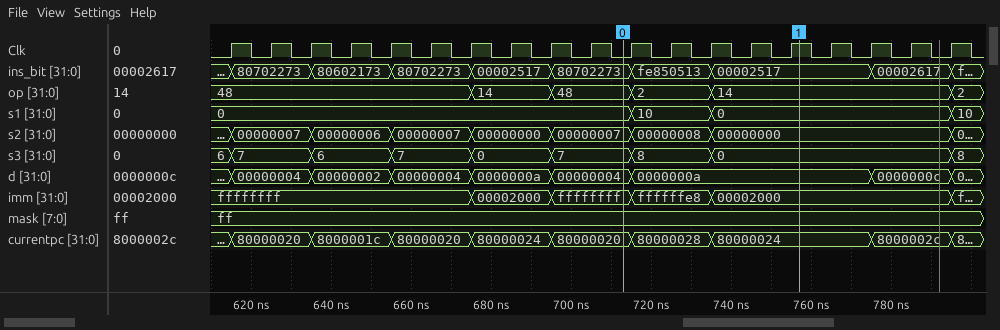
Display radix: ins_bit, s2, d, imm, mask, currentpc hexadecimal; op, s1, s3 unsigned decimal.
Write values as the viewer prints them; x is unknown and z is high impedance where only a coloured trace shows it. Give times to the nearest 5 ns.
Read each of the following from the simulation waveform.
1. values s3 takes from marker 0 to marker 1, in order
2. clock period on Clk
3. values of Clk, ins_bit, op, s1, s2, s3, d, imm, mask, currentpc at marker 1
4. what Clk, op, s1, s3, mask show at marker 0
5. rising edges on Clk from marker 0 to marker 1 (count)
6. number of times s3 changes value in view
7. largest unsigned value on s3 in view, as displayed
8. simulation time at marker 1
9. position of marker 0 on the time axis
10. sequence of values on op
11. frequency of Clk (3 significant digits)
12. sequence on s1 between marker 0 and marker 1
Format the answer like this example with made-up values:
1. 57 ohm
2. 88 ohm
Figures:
1. 7, 8, 0
2. 10 ns
3. Clk=1, ins_bit=00002517, op=14, s1=0, s2=00000000, s3=0, d=0000000a, imm=00002000, mask=ff, currentpc=80000024
4. Clk=0, op=48, s1=0, s3=7, mask=ff
5. 5
6. 8
7. 8
8. 755 ns
9. 715 ns
10. 48, 14, 48, 2, 14, 2
11. 100 MHz
12. 0, 10, 0
